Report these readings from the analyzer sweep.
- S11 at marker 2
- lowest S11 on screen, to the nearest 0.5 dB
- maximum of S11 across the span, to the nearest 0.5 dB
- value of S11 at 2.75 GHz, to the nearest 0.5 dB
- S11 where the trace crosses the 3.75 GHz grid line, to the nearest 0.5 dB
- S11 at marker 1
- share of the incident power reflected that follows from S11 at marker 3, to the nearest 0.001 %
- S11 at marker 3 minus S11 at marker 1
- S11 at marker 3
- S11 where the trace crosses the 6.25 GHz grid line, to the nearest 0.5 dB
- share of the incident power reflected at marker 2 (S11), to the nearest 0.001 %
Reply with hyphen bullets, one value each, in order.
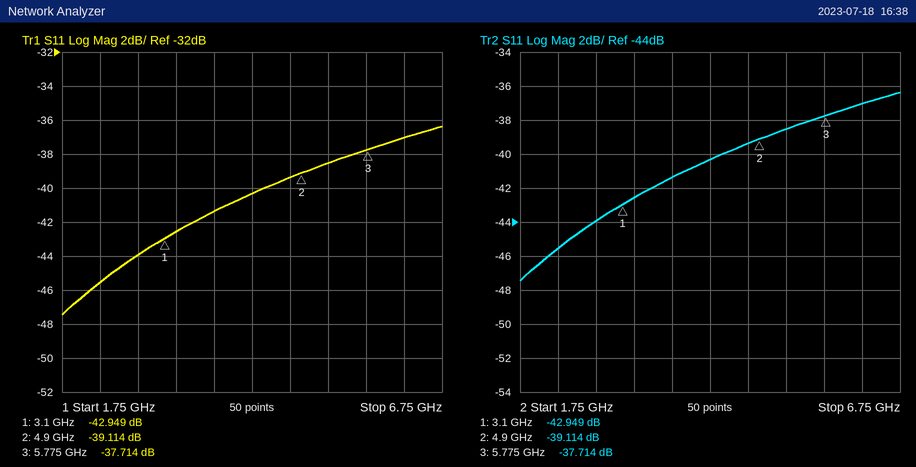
- -39.114 dB
- -47.5 dB
- -36.5 dB
- -44.0 dB
- -41.5 dB
- -42.949 dB
- 0.017 %
- 5.235 dB
- -37.714 dB
- -37.0 dB
- 0.012 %
